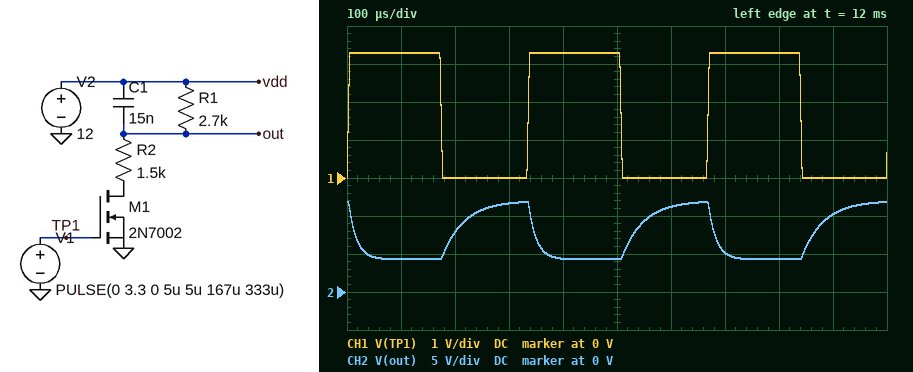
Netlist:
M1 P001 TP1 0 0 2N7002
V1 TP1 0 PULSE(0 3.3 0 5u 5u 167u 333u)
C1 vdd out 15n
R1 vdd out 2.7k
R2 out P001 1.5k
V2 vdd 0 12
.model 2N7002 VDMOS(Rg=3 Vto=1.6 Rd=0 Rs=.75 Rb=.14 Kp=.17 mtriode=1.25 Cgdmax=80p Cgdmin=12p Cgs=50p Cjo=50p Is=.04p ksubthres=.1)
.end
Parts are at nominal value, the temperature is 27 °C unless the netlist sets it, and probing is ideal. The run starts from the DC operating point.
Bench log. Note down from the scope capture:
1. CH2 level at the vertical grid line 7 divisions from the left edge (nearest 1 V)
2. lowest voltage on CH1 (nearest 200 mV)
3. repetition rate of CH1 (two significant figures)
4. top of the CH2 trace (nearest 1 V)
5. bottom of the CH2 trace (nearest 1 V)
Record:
5 V
0 V
3.0 kHz
12 V
4 V
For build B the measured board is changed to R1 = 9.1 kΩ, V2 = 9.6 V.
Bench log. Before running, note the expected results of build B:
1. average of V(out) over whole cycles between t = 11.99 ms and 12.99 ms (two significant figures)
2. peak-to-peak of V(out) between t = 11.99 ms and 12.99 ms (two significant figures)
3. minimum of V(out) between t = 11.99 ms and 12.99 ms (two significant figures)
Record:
3.3 V
5.7 V
1.4 V
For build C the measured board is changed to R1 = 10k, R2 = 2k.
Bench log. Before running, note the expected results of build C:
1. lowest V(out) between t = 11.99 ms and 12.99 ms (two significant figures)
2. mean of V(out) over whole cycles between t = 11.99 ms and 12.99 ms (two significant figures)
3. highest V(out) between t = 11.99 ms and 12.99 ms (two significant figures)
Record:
2.0 V
4.4 V
8.6 V
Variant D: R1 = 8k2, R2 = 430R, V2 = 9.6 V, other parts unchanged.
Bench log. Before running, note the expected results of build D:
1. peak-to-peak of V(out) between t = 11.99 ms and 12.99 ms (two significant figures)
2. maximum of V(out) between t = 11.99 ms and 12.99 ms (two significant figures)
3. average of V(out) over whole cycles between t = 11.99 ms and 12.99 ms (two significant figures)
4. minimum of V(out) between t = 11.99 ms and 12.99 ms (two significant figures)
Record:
6.6 V
7.1 V
2.6 V
480 mV
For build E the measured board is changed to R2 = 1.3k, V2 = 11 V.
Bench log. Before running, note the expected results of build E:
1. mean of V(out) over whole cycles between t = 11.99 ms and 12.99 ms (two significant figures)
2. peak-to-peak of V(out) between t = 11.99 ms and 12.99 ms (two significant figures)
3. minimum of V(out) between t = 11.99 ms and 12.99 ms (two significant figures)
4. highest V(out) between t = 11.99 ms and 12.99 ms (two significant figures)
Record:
6.6 V
7.3 V
3.6 V
11 V
